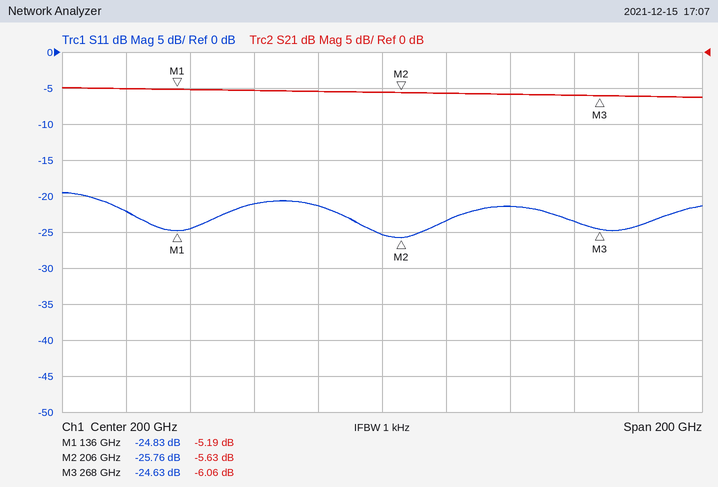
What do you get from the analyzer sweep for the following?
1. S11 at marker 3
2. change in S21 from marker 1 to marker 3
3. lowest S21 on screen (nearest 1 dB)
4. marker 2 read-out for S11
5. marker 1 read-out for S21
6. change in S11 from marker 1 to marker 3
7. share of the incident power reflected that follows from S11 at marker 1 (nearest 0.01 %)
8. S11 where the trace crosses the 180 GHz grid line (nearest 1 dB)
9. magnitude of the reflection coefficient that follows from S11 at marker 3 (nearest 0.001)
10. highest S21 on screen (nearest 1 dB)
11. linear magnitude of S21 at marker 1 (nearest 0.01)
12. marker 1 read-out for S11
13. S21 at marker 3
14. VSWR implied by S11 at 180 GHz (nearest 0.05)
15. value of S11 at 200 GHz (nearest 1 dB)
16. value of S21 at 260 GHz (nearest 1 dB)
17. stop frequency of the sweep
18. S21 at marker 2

-24.63 dB
-0.87 dB
-6 dB
-25.76 dB
-5.19 dB
0.20 dB
0.33 %
-21 dB
0.059
-5 dB
0.55
-24.83 dB
-6.06 dB
1.20
-25 dB
-6 dB
300 GHz
-5.63 dB
